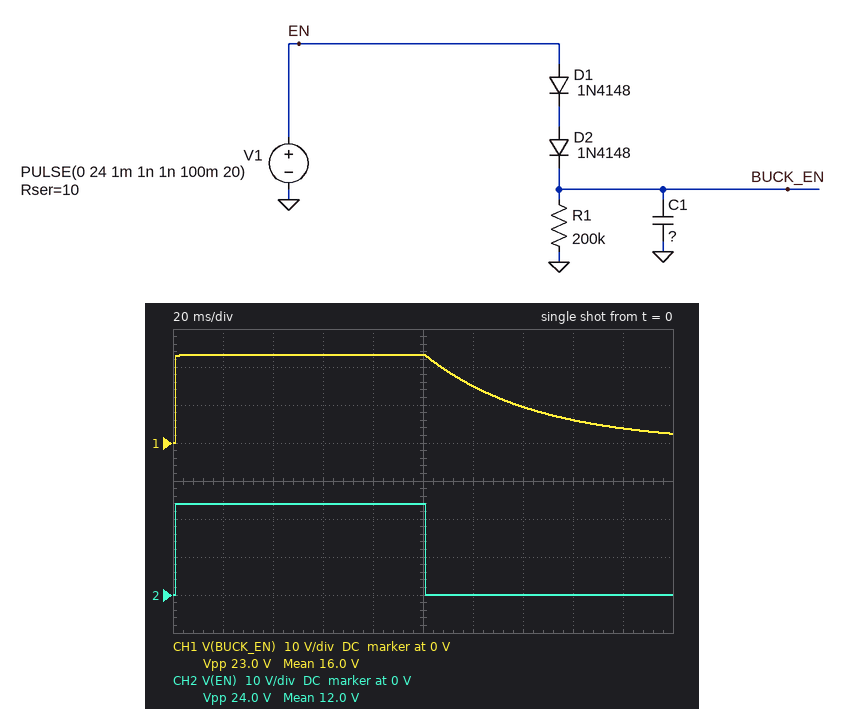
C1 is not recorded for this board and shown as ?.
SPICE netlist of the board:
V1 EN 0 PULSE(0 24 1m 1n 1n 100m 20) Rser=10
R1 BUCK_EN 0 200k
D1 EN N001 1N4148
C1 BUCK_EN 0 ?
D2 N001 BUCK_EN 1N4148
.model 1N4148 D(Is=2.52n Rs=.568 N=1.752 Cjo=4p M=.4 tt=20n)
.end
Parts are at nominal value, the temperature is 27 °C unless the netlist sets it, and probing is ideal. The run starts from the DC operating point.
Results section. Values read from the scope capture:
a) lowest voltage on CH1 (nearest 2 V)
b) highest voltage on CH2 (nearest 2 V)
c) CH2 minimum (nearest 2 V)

0 V
24 V
0 V
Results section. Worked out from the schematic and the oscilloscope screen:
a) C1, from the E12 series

220 nF
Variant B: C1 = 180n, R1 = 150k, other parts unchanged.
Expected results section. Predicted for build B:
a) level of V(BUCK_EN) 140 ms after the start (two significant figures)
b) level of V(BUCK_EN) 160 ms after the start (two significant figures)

5.4 V
2.6 V
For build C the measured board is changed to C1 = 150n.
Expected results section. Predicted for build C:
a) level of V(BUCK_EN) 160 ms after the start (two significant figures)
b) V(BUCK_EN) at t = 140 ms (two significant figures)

3.2 V
6.3 V
